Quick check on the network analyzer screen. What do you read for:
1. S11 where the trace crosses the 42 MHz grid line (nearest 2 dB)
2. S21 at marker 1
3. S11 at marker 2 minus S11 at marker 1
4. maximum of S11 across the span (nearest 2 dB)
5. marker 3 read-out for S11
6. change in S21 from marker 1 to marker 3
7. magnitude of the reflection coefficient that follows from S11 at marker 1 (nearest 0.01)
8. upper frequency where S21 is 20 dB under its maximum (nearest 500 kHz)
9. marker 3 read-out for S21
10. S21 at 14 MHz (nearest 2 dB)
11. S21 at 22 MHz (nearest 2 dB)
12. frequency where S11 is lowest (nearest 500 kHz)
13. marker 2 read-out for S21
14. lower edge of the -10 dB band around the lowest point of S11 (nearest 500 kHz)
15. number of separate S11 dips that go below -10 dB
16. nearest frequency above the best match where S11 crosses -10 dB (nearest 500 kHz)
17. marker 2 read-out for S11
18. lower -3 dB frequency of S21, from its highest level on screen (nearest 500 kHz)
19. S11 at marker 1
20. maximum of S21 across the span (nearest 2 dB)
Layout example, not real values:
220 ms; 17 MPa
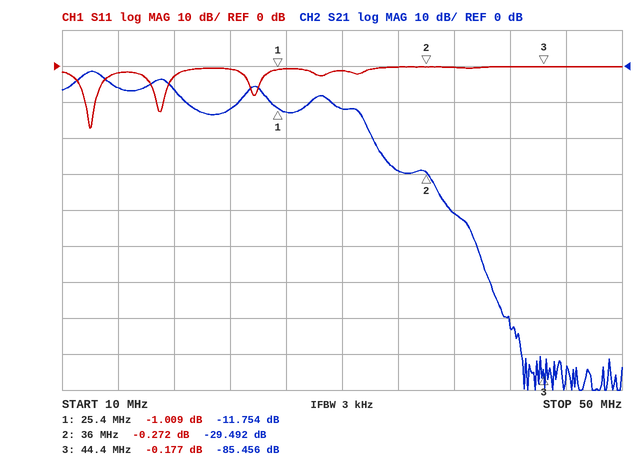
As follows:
0 dB; -11.754 dB; 0.737 dB; 0 dB; -0.177 dB; -73.702 dB; 0.89; 32.5 MHz; -85.456 dB; -6 dB; -12 dB; 12.0 MHz; -29.492 dB; 11.5 MHz; 2; 12.5 MHz; -0.272 dB; 11.0 MHz; -1.009 dB; -2 dB
